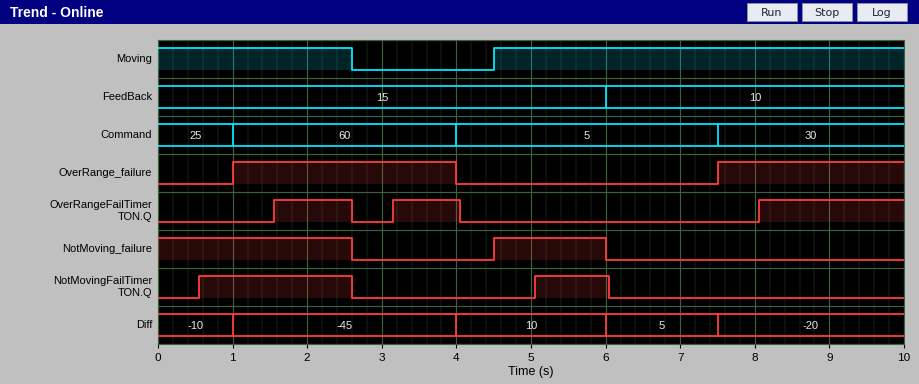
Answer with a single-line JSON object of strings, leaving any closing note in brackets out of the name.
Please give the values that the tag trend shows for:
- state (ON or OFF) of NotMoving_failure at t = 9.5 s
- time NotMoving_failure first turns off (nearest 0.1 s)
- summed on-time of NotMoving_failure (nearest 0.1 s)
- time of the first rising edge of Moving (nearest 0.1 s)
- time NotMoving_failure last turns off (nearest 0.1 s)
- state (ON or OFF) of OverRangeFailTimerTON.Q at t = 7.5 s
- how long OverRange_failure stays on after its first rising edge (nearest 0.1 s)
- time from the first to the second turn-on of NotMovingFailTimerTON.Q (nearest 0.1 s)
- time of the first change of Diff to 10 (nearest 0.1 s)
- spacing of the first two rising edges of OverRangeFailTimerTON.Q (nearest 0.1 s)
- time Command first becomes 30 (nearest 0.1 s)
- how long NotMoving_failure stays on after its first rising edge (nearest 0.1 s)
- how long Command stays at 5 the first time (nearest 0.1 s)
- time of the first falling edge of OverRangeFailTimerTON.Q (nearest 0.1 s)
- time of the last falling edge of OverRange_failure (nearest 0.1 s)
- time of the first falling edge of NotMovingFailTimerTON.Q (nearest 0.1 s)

{"state (ON or OFF) of NotMoving_failure at t = 9.5 s": "OFF", "time NotMoving_failure first turns off": "2.6 s", "summed on-time of NotMoving_failure": "4.1 s", "time of the first rising edge of Moving": "4.5 s", "time NotMoving_failure last turns off": "6.0 s", "state (ON or OFF) of OverRangeFailTimerTON.Q at t = 7.5 s": "OFF", "how long OverRange_failure stays on after its first rising edge": "3.0 s", "time from the first to the second turn-on of NotMovingFailTimerTON.Q": "4.5 s", "time of the first change of Diff to 10": "4.0 s", "spacing of the first two rising edges of OverRangeFailTimerTON.Q": "1.6 s", "time Command first becomes 30": "7.5 s", "how long NotMoving_failure stays on after its first rising edge": "1.5 s", "how long Command stays at 5 the first time": "3.5 s", "time of the first falling edge of OverRangeFailTimerTON.Q": "2.6 s", "time of the last falling edge of OverRange_failure": "4.0 s", "time of the first falling edge of NotMovingFailTimerTON.Q": "2.6 s"}
